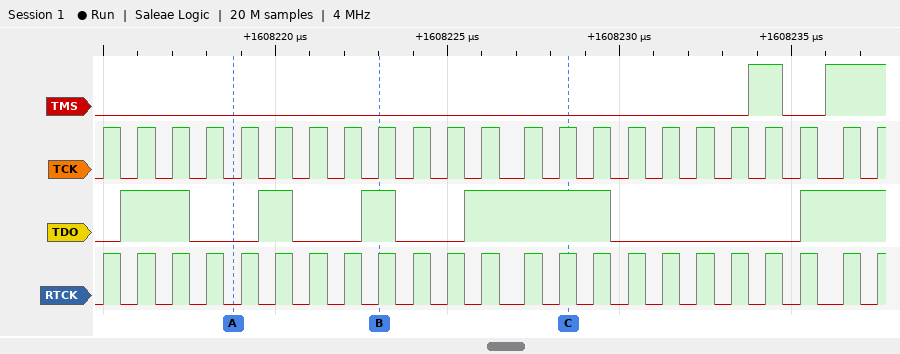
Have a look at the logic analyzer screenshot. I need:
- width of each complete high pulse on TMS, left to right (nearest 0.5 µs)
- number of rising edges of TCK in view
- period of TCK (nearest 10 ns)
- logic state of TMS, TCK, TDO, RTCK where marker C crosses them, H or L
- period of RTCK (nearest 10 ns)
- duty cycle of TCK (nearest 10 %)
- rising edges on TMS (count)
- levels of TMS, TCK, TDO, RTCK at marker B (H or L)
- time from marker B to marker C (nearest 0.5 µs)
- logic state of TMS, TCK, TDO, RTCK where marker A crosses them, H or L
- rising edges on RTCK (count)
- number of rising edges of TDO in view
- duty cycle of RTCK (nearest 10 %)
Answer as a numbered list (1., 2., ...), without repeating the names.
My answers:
1. 1 µs
2. 23
3. 1020 ns
4. TMS=L, TCK=H, TDO=H, RTCK=H
5. 1020 ns
6. 50 %
7. 2
8. TMS=L, TCK=H, TDO=H, RTCK=H
9. 5.5 µs
10. TMS=L, TCK=L, TDO=L, RTCK=L
11. 23
12. 5
13. 50 %
